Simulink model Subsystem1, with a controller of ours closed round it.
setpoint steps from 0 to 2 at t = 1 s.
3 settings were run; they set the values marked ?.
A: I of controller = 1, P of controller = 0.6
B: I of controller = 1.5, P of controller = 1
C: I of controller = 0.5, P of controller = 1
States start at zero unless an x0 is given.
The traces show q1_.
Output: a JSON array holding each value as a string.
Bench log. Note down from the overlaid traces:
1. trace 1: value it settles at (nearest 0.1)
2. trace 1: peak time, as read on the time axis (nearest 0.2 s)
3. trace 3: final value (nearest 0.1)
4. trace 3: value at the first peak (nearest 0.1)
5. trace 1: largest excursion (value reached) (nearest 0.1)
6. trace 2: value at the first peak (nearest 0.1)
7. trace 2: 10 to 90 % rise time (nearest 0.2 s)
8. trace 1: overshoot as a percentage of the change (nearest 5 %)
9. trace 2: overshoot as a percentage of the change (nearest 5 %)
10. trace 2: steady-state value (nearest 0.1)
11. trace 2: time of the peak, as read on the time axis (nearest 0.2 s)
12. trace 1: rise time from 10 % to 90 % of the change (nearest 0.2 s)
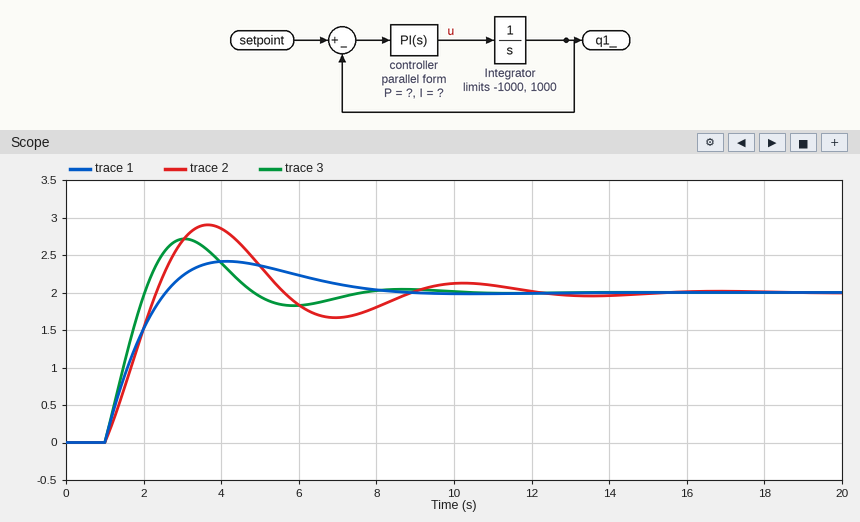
["2.0", "4.2 s", "2.0", "2.7", "2.4", "2.9", "1.0 s", "20 %", "45 %", "2.0", "3.6 s", "1.2 s"]
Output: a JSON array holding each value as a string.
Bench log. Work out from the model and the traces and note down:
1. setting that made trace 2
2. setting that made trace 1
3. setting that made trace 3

["A", "C", "B"]
